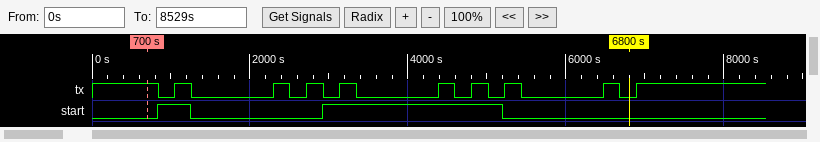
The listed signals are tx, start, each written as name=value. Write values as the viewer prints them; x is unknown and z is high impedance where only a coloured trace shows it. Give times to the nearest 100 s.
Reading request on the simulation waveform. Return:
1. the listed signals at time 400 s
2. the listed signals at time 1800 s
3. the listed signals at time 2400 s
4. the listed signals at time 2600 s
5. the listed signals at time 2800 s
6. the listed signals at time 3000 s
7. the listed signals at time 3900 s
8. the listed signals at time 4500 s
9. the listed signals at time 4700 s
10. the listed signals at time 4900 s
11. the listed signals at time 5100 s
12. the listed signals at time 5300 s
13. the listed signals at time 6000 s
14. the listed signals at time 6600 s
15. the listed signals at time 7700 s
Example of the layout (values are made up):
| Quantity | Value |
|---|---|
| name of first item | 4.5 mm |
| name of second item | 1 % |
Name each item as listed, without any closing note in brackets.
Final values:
| Quantity | Value |
|---|---|
| the listed signals at time 400 s | tx=1, start=0 |
| the listed signals at time 1800 s | tx=0, start=0 |
| the listed signals at time 2400 s | tx=1, start=0 |
| the listed signals at time 2600 s | tx=0, start=0 |
| the listed signals at time 2800 s | tx=1, start=0 |
| the listed signals at time 3000 s | tx=0, start=1 |
| the listed signals at time 3900 s | tx=0, start=1 |
| the listed signals at time 4500 s | tx=1, start=1 |
| the listed signals at time 4700 s | tx=0, start=1 |
| the listed signals at time 4900 s | tx=1, start=1 |
| the listed signals at time 5100 s | tx=0, start=1 |
| the listed signals at time 5300 s | tx=1, start=0 |
| the listed signals at time 6000 s | tx=0, start=0 |
| the listed signals at time 6600 s | tx=1, start=0 |
| the listed signals at time 7700 s | tx=1, start=0 |
